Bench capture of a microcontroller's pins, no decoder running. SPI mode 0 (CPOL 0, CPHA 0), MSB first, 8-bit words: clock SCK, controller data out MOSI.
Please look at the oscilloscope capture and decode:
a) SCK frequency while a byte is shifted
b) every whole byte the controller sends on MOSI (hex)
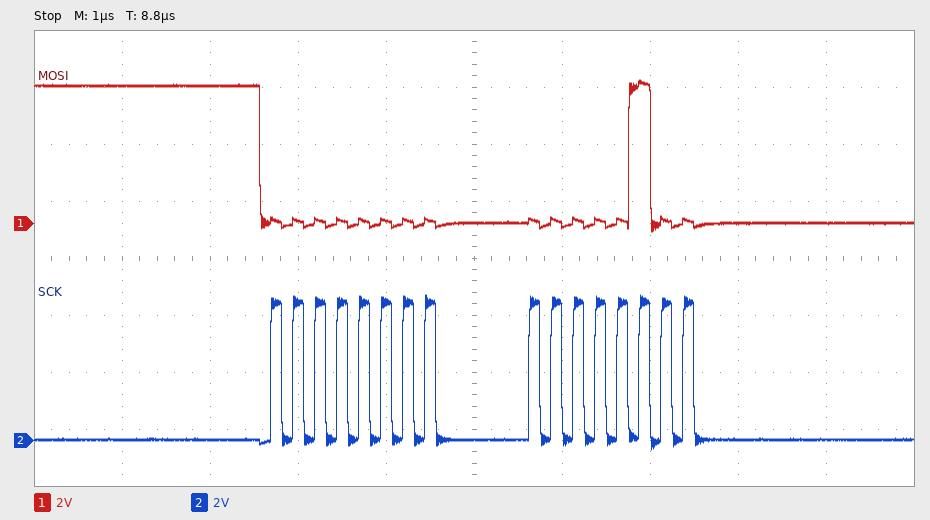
4 MHz
0x00 0x04
